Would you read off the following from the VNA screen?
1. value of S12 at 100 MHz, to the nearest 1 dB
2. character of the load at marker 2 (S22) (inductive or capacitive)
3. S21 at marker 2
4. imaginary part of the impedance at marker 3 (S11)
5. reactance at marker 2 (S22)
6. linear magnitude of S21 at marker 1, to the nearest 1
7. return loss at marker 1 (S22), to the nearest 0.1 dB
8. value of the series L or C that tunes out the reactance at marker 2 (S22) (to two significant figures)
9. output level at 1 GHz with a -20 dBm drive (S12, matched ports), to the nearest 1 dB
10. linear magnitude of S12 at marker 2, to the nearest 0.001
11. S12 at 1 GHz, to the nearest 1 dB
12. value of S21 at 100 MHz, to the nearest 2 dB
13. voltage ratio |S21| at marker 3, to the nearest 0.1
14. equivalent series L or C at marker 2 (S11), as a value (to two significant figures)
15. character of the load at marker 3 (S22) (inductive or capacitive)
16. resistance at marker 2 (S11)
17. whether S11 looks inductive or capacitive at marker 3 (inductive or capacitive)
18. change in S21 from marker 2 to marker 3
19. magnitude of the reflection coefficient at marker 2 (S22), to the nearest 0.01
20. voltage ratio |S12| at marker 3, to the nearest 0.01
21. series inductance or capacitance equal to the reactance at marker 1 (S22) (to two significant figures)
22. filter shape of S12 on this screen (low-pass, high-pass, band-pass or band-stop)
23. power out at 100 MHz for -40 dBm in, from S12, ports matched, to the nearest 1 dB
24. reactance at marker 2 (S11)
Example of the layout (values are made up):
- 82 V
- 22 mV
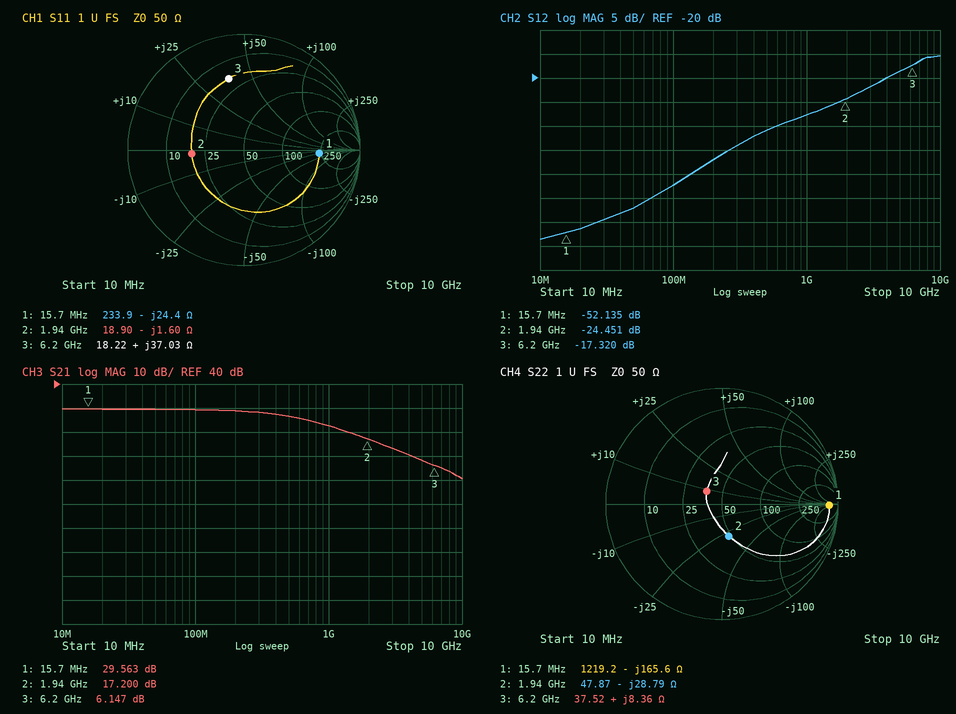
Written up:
- -42 dB
- capacitive
- 17.200 dB
- +37.03 Ω
- -28.79 Ω
- 30
- 0.7 dB
- 2.4 nH
- -48 dBm
- 0.060
- -28 dB
- 30 dB
- 2.0
- 51 pF
- inductive
- 18.90 Ω
- inductive
- -11.053 dB
- 0.28
- 0.14
- 61 pF
- high-pass
- -82 dBm
- -1.60 Ω
